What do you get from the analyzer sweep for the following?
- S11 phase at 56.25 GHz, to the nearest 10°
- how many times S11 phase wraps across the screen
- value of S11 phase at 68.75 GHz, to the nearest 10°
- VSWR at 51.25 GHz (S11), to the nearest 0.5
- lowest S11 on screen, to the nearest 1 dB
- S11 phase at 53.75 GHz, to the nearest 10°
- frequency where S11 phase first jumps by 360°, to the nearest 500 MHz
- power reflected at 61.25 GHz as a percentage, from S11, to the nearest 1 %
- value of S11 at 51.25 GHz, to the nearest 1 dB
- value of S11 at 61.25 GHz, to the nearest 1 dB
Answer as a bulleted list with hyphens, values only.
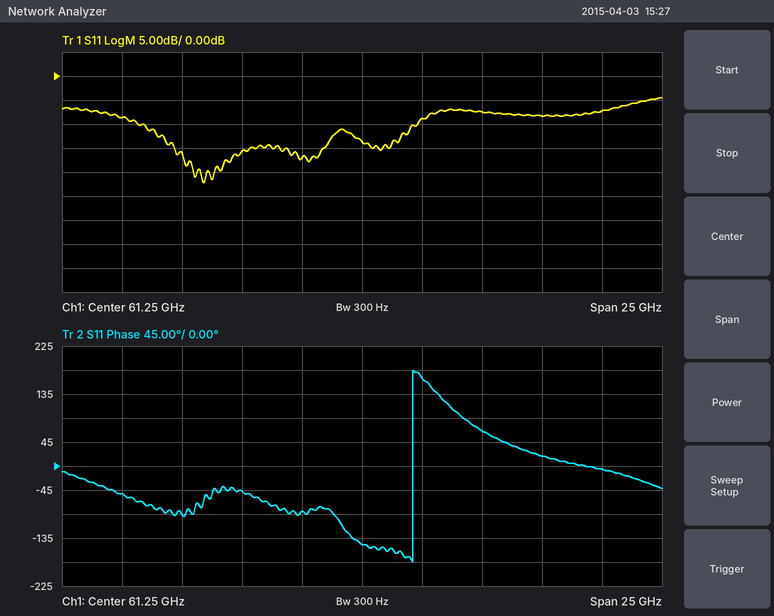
- -50°
- 1
- 20°
- 2.0
- -22 dB
- -90°
- 63.5 GHz
- 4 %
- -9 dB
- -14 dB
